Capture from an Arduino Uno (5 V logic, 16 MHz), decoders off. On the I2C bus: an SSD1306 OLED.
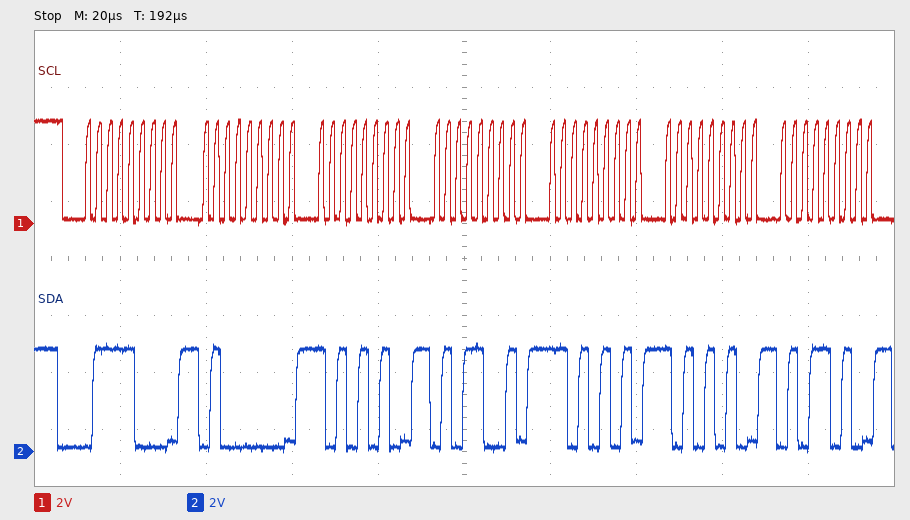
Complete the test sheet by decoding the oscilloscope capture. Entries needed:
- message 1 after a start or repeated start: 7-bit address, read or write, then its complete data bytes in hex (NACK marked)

0x3C write: 40 AA 59 D5 AA 5A
